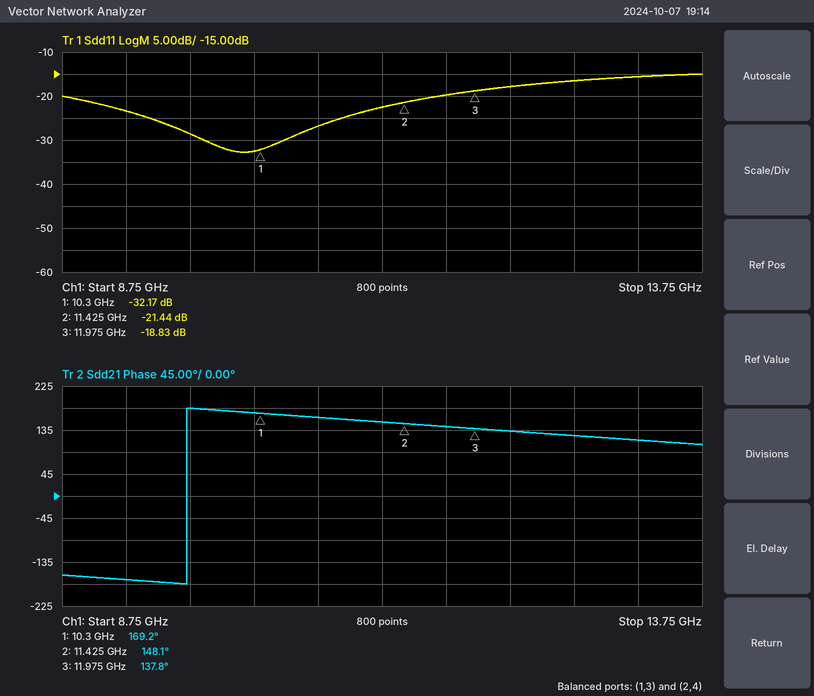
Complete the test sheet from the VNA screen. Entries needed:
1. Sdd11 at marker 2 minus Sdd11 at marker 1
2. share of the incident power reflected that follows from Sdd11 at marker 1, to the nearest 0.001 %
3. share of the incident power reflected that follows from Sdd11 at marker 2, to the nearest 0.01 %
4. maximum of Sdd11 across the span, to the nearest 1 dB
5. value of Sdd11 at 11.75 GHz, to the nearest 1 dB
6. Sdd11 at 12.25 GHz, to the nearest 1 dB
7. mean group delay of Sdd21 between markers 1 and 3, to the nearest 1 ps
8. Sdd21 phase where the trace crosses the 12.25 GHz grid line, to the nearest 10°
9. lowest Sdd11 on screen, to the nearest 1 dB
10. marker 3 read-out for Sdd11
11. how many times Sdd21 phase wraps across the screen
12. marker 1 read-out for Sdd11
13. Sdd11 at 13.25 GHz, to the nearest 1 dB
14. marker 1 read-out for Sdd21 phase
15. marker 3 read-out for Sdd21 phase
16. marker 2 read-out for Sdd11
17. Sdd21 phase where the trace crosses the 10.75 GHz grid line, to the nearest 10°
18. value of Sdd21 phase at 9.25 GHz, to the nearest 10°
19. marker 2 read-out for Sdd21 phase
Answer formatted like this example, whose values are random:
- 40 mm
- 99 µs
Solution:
- 10.73 dB
- 0.061 %
- 0.72 %
- -15 dB
- -20 dB
- -18 dB
- 52 ps
- 130°
- -33 dB
- -18.83 dB
- 1
- -32.17 dB
- -16 dB
- 169.2°
- 137.8°
- -21.44 dB
- 160°
- -170°
- 148.1°
